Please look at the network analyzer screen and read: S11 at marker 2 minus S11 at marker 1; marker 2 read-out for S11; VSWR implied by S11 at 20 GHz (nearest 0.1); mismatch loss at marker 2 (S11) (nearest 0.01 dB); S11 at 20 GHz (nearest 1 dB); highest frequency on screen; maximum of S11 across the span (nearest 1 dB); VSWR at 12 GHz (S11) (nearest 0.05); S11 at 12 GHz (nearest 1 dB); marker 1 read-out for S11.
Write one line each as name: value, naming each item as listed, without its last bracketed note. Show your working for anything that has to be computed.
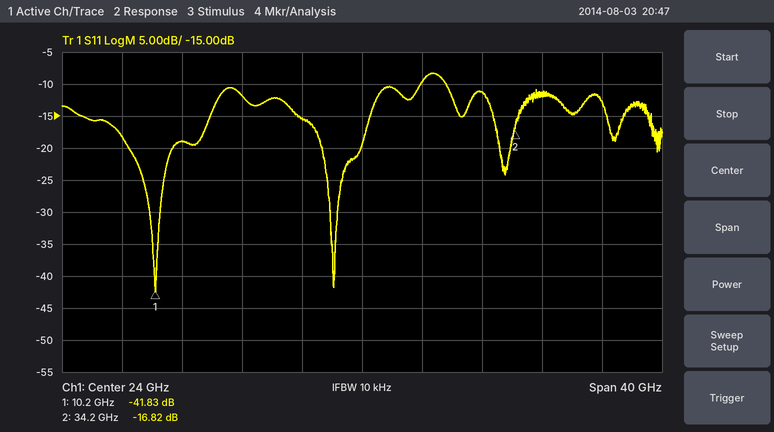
S11 at marker 2 minus S11 at marker 1: -16.82 − (-41.83) = 25.01 dB
marker 2 read-out for S11: -16.82 dB
VSWR implied by S11 at 20 GHz: |Γ| = 10^(-15/20) = 0.1778; VSWR = (1 + 0.1778)/(1 − 0.1778) ≈ 1.4
mismatch loss at marker 2 (S11): −10 log10(1 − 10^(-16.82/10)) ≈ 0.09 dB
S11 at 20 GHz: -15 dB
highest frequency on screen: 44 GHz
maximum of S11 across the span: -8 dB
VSWR at 12 GHz (S11): |Γ| = 10^(-19/20) = 0.1122; VSWR = (1 + 0.1122)/(1 − 0.1122) ≈ 1.25
S11 at 12 GHz: -19 dB
marker 1 read-out for S11: -41.83 dB
